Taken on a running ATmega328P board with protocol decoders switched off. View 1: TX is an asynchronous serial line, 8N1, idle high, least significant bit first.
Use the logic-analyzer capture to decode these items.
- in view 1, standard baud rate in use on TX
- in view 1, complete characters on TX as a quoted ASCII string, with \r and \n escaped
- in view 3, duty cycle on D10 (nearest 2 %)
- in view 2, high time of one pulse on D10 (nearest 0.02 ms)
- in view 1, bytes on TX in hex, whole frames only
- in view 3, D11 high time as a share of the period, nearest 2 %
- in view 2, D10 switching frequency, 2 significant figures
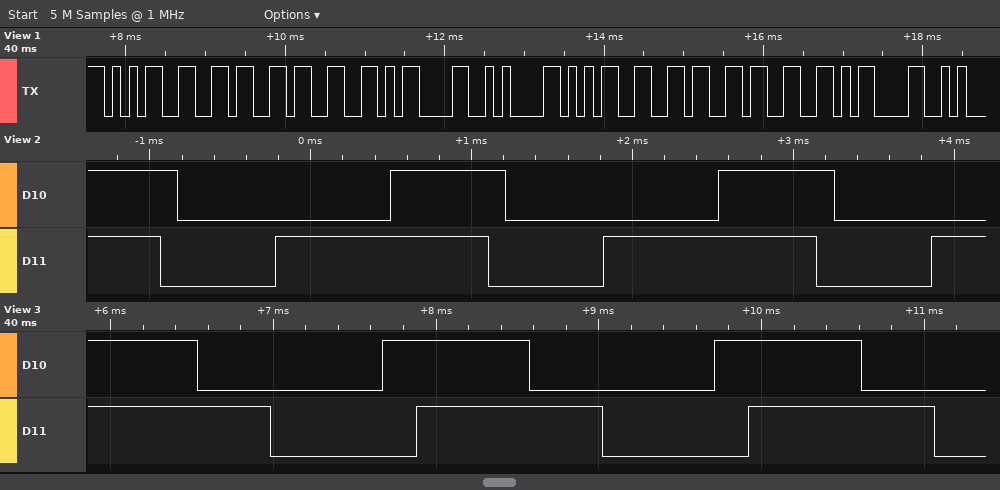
9600 baud
"563\r\n563\r"
44 %
0.72 ms
0x35 0x36 0x33 0x0D 0x0A 0x35 0x36 0x33 0x0D
56 %
490 Hz
